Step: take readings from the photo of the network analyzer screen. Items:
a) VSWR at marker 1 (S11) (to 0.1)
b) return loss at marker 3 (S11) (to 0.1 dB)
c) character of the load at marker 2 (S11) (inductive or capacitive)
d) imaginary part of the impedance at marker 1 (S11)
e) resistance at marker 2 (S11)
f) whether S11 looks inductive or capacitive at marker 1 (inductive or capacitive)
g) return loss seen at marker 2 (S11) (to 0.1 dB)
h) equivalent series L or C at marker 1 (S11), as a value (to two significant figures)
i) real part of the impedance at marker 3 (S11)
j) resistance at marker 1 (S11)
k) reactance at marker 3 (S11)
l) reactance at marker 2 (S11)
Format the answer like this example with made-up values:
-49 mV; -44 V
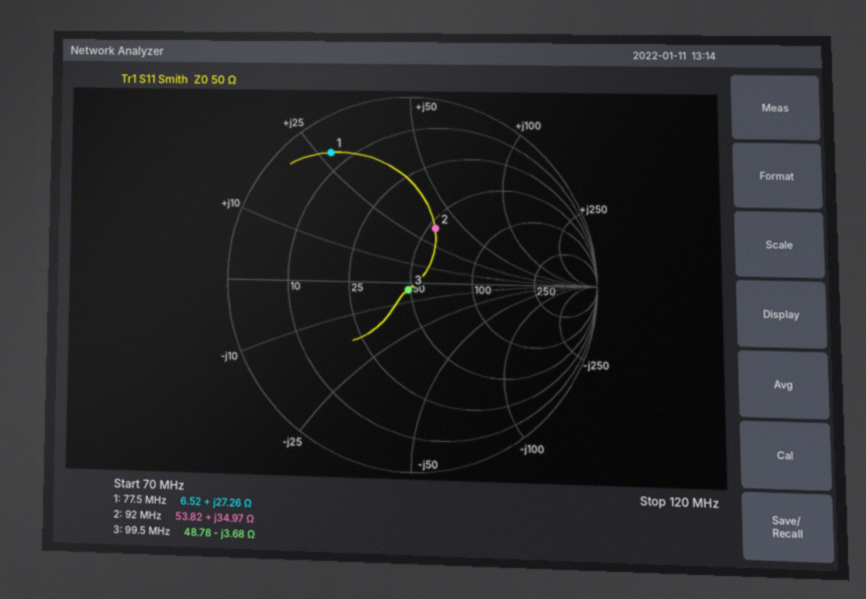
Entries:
10.0; 28.1 dB; inductive; +27.26 Ω; 53.82 Ω; inductive; 9.9 dB; 56 nH; 48.78 Ω; 6.52 Ω; -3.68 Ω; +34.97 Ω
